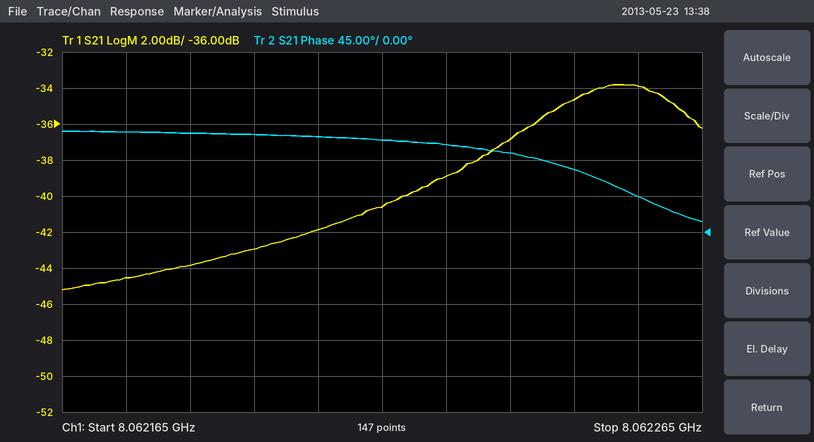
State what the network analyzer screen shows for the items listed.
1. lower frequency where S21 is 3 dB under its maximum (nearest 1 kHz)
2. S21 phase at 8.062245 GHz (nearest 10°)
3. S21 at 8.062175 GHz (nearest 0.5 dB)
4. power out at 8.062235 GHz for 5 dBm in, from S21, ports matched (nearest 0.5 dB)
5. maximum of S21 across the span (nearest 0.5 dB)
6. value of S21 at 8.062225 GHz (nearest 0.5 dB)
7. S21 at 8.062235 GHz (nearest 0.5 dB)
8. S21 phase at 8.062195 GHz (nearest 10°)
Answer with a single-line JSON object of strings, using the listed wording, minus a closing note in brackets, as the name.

{"lower frequency where S21 is 3 dB under its maximum": "8.062235 GHz", "S21 phase at 8.062245 GHz": "80°", "S21 at 8.062175 GHz": "-44.5 dB", "power out at 8.062235 GHz for 5 dBm in, from S21, ports matched": "-32.0 dBm", "maximum of S21 across the span": "-34.0 dB", "value of S21 at 8.062225 GHz": "-39.0 dB", "S21 at 8.062235 GHz": "-37.0 dB", "S21 phase at 8.062195 GHz": "120°"}
